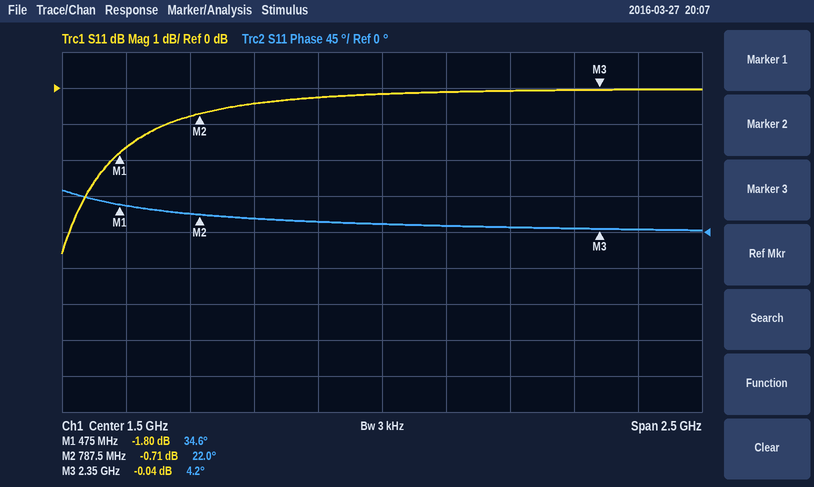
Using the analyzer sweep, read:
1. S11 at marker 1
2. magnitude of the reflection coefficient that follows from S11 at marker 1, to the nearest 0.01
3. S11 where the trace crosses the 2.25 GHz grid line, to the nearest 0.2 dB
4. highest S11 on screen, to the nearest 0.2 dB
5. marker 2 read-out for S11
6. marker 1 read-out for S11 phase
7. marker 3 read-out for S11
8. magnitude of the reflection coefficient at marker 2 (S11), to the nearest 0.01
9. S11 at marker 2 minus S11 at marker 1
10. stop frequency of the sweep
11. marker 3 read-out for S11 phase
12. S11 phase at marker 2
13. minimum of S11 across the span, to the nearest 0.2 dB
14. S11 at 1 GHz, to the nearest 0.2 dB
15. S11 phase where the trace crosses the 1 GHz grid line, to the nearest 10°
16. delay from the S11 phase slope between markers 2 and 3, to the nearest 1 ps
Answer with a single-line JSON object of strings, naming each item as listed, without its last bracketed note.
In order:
{"S11 at marker 1": "-1.80 dB", "magnitude of the reflection coefficient that follows from S11 at marker 1, to the nearest 0.01": "0.81", "S11 where the trace crosses the 2.25 GHz grid line, to the nearest 0.2 dB": "0.0 dB", "highest S11 on screen, to the nearest 0.2 dB": "0.0 dB", "marker 2 read-out for S11": "-0.71 dB", "marker 1 read-out for S11 phase": "34.6°", "marker 3 read-out for S11": "-0.04 dB", "magnitude of the reflection coefficient at marker 2 (S11), to the nearest 0.01": "0.92", "S11 at marker 2 minus S11 at marker 1": "1.09 dB", "stop frequency of the sweep": "2.75 GHz", "marker 3 read-out for S11 phase": "4.2°", "S11 phase at marker 2": "22.0°", "minimum of S11 across the span, to the nearest 0.2 dB": "-4.6 dB", "S11 at 1 GHz, to the nearest 0.2 dB": "-0.4 dB", "S11 phase where the trace crosses the 1 GHz grid line, to the nearest 10°": "20°", "delay from the S11 phase slope between markers 2 and 3, to the nearest 1 ps": "32 ps"}
